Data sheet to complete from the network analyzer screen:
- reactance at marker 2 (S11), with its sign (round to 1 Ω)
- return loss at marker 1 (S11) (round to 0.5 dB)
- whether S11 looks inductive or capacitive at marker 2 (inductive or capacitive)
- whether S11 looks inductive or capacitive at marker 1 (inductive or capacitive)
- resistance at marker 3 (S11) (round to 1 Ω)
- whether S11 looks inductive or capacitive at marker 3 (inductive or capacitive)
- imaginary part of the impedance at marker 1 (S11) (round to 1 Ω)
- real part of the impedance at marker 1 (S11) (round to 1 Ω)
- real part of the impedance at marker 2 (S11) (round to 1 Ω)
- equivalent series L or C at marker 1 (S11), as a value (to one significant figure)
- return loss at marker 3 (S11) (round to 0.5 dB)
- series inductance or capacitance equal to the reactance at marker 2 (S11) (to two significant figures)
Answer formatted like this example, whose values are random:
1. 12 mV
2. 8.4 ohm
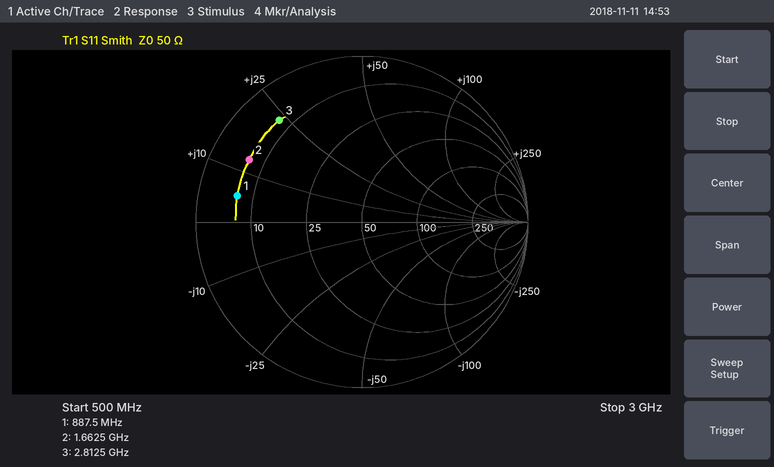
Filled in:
1. +13 Ω
2. 2.5 dB
3. inductive
4. inductive
5. 7 Ω
6. inductive
7. +5 Ω
8. 7 Ω
9. 7 Ω
10. 900 pH
11. 2.0 dB
12. 1.2 nH
